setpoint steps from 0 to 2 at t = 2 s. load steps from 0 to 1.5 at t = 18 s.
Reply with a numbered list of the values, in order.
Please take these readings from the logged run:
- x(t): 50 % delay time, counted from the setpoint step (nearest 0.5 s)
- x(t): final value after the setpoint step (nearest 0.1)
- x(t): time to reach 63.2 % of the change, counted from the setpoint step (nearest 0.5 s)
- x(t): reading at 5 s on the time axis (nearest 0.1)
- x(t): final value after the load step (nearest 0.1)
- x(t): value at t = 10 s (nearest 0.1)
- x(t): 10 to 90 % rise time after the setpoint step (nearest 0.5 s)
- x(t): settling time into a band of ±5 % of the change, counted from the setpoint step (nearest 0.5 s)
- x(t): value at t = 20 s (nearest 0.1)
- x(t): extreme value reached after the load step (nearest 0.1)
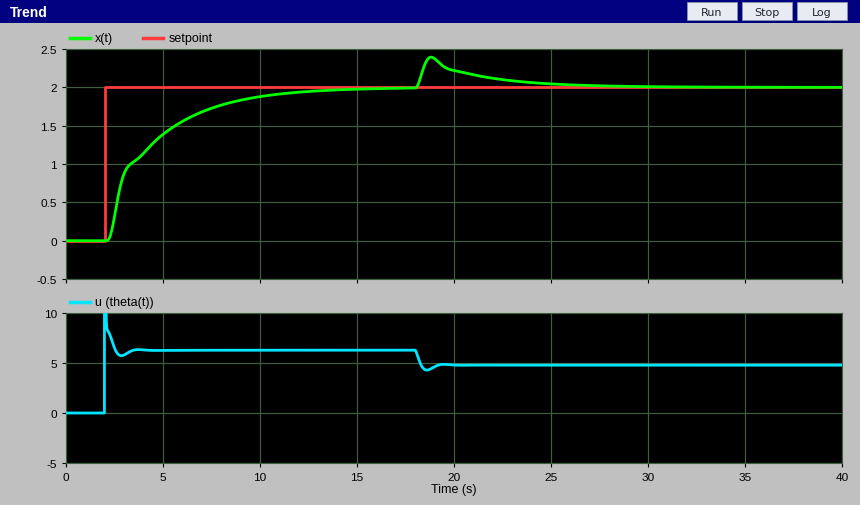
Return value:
1. 1.5 s
2. 2.0
3. 2.5 s
4. 1.4
5. 2.0
6. 1.9
7. 6.0 s
8. 8.5 s
9. 2.2
10. 2.4
